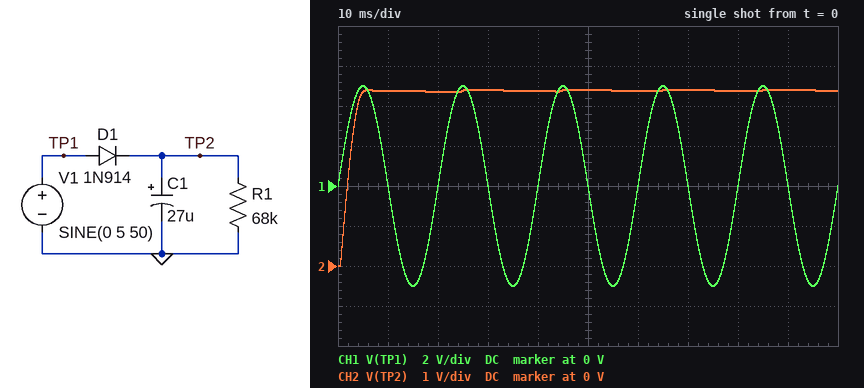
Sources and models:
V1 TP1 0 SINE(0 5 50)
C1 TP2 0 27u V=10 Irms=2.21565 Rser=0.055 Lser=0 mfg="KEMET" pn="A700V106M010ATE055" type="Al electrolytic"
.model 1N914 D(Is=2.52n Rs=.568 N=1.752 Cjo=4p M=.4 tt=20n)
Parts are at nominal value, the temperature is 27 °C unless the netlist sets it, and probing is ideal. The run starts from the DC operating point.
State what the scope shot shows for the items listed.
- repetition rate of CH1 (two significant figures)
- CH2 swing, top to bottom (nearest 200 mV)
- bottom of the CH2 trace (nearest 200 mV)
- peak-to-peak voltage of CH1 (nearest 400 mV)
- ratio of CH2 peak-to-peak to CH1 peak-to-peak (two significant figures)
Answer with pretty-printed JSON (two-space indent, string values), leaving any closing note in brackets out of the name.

{
  "repetition rate of CH1": "50 Hz",
  "CH2 swing, top to bottom": "4.4 V",
  "bottom of the CH2 trace": "0 V",
  "peak-to-peak voltage of CH1": "10.0 V",
  "ratio of CH2 peak-to-peak to CH1 peak-to-peak": "0.44"
}
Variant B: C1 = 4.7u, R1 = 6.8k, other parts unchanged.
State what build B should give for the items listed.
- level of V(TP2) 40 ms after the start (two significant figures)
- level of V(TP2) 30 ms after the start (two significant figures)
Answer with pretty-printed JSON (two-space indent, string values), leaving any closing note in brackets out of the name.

{
  "level of V(TP2) 40 ms after the start": "2.8 V",
  "level of V(TP2) 30 ms after the start": "3.8 V"
}
